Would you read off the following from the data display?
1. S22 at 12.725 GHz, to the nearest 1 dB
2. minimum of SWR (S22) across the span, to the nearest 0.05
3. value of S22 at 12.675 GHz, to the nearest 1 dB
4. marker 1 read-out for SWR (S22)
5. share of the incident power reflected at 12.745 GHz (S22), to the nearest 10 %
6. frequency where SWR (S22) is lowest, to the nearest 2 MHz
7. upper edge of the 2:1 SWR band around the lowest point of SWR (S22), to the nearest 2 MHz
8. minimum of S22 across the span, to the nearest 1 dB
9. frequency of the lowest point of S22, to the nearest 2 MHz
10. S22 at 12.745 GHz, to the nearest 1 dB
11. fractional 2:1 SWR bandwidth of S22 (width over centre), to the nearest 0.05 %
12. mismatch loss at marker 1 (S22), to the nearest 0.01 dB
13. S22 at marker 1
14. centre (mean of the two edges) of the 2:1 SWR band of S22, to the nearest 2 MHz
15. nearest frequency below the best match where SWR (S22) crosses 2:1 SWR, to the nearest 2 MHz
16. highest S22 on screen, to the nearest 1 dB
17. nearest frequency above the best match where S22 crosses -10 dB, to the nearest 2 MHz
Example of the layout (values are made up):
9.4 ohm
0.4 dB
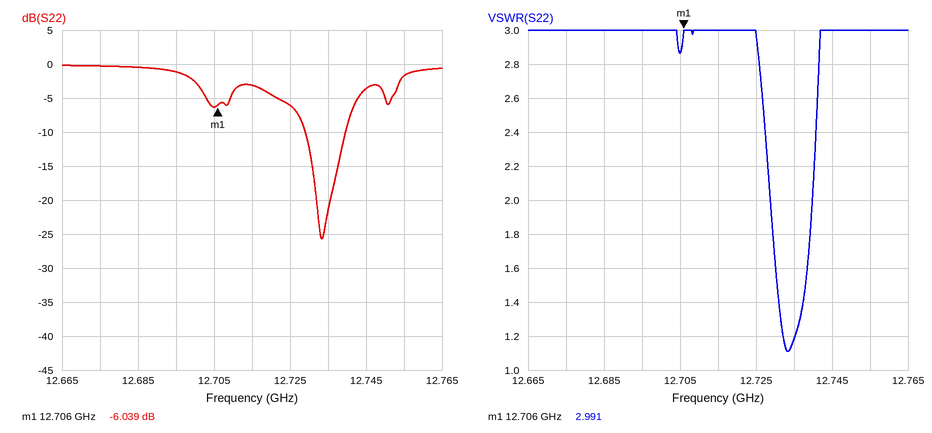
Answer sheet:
-6 dB
1.10
0 dB
2.991
40 %
12.734 GHz
12.740 GHz
-26 dB
12.734 GHz
-4 dB
0.10 %
1.24 dB
-6.039 dB
12.734 GHz
12.728 GHz
0 dB
12.740 GHz
